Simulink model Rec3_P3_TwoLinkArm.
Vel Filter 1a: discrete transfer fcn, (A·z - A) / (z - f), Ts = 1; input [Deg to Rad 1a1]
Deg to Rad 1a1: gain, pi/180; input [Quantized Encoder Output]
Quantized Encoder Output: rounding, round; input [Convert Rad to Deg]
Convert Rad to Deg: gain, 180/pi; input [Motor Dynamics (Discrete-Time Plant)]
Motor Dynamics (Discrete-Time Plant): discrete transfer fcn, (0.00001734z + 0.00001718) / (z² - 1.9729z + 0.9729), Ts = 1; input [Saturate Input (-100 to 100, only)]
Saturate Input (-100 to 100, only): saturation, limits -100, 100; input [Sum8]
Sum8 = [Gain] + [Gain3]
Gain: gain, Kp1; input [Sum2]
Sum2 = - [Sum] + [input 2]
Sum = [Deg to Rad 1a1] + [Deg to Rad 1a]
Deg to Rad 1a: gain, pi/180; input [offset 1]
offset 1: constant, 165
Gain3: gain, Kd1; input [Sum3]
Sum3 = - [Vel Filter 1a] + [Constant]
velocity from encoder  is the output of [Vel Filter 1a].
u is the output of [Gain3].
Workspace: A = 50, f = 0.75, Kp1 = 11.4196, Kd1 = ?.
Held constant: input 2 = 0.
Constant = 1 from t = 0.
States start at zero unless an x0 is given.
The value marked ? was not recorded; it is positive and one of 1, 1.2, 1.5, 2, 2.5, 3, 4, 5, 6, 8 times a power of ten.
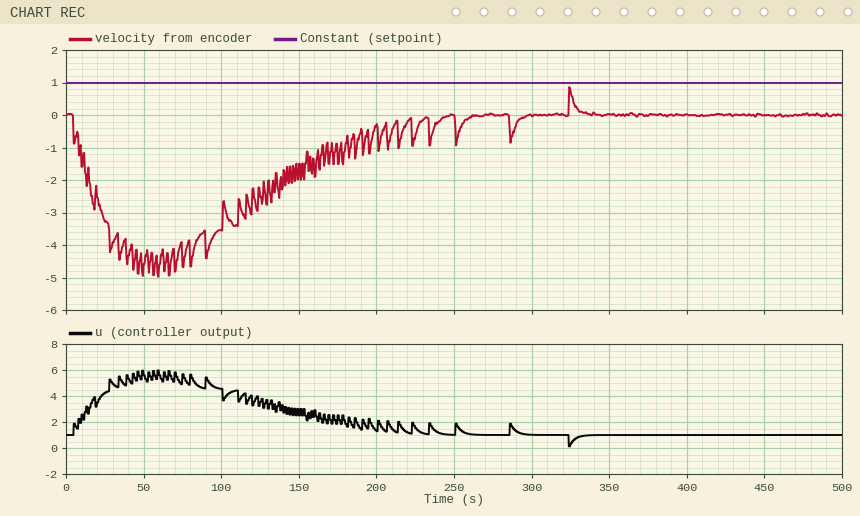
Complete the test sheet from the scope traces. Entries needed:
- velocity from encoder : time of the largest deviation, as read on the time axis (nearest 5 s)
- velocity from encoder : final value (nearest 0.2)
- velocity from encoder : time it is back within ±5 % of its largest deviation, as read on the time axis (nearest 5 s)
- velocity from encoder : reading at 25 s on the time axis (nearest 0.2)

60 s
0.0
330 s
-3.2
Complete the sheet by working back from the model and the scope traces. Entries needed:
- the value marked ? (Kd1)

1
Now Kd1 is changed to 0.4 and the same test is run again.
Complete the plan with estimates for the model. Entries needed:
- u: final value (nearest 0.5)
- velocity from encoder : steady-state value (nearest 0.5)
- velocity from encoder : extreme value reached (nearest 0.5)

0.5
0.0
-5.5
